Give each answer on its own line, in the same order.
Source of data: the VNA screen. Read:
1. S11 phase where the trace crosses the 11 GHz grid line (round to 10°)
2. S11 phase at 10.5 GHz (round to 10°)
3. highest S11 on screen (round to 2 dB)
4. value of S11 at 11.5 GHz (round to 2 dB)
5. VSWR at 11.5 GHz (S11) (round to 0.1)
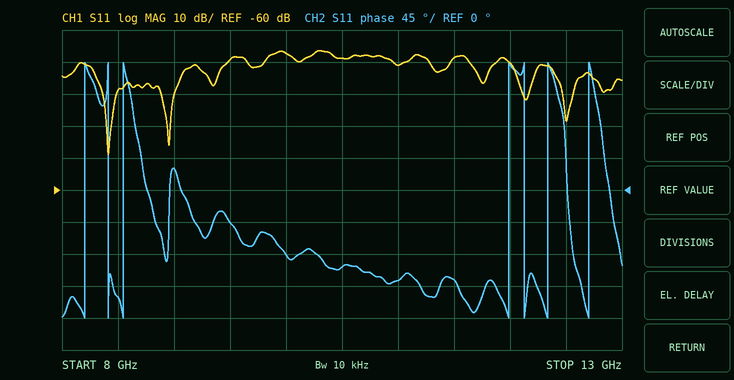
-130°
-110°
-16 dB
-18 dB
1.3
